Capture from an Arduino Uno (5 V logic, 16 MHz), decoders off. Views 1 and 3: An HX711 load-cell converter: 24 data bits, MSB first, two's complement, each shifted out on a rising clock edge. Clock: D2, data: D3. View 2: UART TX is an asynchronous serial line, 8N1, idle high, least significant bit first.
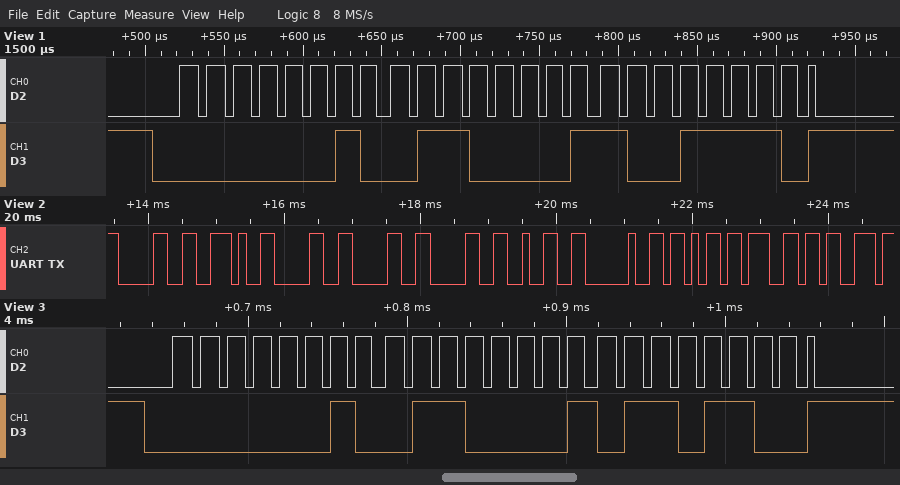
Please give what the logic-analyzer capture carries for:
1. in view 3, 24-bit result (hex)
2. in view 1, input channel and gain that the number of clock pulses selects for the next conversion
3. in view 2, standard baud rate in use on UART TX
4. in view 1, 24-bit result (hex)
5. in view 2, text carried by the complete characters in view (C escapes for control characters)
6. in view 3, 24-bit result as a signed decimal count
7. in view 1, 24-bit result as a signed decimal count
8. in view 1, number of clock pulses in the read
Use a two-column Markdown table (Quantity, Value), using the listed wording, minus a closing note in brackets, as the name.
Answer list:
| Quantity | Value |
|---|---|
| in view 3, 24-bit result | 0x02616C |
| in view 1, input channel and gain that the number of clock pulses selects for the next conversion | channel A, gain 128 |
| in view 2, standard baud rate in use on UART TX | 9600 baud |
| in view 1, 24-bit result | 0x02619E |
| in view 2, text carried by the complete characters in view | "0.0002 kgs" |
| in view 3, 24-bit result as a signed decimal count | 156012 |
| in view 1, 24-bit result as a signed decimal count | 156062 |
| in view 1, number of clock pulses in the read | 25 |
